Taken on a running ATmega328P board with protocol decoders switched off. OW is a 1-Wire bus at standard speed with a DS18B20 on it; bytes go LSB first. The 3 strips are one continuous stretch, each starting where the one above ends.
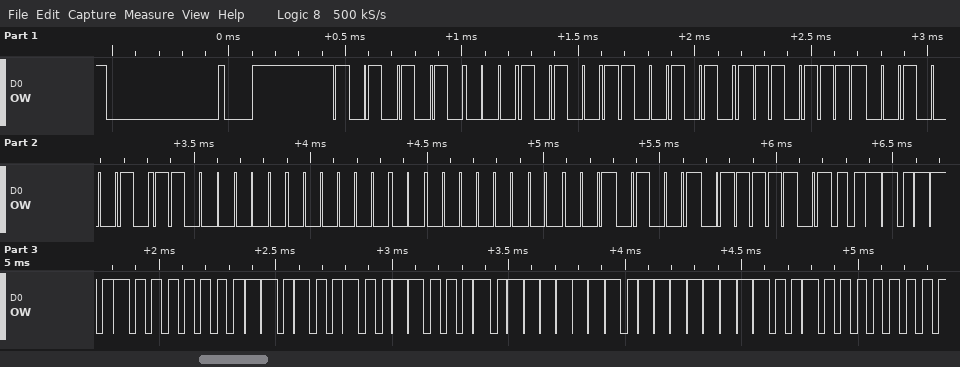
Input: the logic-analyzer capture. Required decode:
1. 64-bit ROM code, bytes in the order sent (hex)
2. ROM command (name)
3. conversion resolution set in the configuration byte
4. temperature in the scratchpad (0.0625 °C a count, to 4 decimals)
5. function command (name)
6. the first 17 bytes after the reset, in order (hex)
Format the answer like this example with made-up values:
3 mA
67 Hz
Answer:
28 53 F7 44 03 00 00 94
Match ROM
12 bits
22.7500 °C
Read Scratchpad
55 28 53 F7 44 03 00 00 94 BE 6C 01 4B 46 7F FF 04
